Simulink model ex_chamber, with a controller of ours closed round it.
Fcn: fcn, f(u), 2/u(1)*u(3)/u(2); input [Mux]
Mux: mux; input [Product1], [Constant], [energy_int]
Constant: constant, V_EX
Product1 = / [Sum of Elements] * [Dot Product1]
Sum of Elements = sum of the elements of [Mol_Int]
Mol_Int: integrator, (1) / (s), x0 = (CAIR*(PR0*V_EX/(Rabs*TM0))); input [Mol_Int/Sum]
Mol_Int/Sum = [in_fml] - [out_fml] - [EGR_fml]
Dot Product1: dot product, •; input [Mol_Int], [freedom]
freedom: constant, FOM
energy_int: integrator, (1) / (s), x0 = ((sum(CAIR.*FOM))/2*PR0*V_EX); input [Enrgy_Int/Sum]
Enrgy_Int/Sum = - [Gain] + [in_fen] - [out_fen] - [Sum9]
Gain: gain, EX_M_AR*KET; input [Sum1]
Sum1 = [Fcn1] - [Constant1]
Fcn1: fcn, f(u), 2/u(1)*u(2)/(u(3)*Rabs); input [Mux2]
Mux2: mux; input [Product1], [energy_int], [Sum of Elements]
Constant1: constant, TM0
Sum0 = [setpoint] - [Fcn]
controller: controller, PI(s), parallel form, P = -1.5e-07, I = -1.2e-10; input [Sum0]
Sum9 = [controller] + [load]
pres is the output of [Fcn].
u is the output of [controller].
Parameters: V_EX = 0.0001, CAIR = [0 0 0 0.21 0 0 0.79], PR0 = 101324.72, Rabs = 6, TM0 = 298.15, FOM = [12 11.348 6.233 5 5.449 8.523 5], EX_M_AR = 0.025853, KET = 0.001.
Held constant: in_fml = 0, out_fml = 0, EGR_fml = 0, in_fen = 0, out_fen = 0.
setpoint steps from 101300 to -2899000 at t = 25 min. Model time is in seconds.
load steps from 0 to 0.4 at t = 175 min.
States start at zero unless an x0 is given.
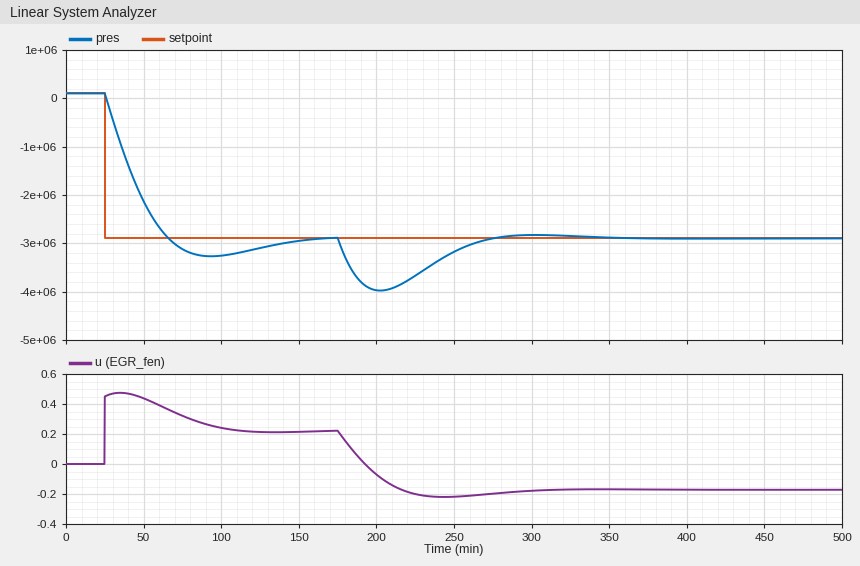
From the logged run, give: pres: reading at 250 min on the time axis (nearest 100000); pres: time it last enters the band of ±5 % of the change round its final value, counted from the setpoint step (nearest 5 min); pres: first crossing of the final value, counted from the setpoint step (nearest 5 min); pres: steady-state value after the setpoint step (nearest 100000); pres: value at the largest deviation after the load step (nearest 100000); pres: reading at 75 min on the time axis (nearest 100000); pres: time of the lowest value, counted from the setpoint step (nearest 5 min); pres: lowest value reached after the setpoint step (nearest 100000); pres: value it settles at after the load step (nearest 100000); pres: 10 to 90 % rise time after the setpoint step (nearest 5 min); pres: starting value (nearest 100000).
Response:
-3200000
105 min
40 min
-2900000
-4000000
-3100000
70 min
-3300000
-2900000
30 min
100000
